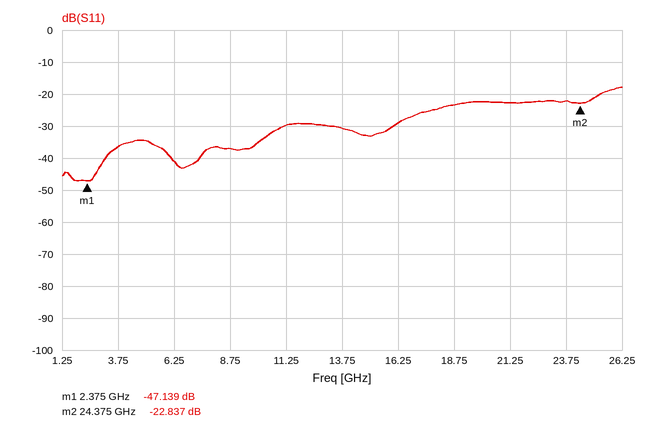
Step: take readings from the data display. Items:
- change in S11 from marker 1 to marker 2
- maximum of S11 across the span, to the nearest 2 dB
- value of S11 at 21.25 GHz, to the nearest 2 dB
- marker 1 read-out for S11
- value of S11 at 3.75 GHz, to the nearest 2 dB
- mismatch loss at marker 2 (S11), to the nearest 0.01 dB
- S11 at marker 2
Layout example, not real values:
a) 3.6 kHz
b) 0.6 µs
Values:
a) 24.302 dB
b) -18 dB
c) -22 dB
d) -47.139 dB
e) -36 dB
f) 0.02 dB
g) -22.837 dB
